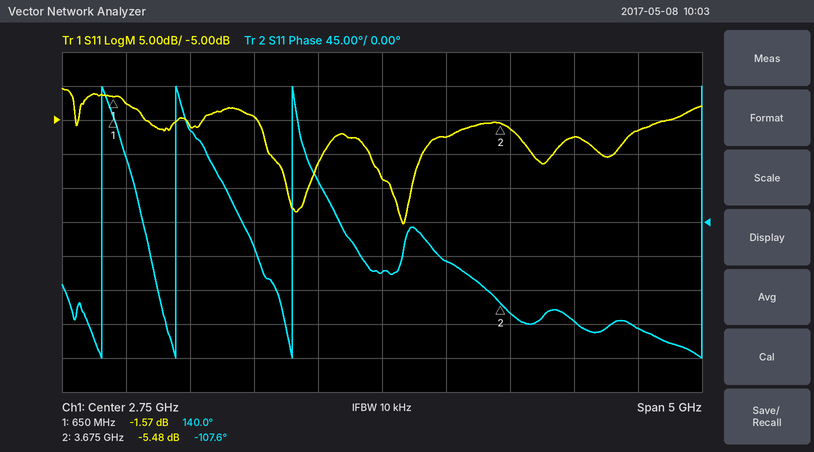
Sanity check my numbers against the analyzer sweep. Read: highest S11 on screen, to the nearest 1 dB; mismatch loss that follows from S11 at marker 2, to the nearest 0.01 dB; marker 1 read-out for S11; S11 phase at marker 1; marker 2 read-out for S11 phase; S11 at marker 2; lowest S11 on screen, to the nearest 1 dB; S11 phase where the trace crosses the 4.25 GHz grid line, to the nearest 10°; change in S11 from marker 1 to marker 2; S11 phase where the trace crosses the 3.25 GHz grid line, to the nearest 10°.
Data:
0 dB
1.45 dB
-1.57 dB
140.0°
-107.6°
-5.48 dB
-20 dB
-130°
-3.91 dB
-50°
